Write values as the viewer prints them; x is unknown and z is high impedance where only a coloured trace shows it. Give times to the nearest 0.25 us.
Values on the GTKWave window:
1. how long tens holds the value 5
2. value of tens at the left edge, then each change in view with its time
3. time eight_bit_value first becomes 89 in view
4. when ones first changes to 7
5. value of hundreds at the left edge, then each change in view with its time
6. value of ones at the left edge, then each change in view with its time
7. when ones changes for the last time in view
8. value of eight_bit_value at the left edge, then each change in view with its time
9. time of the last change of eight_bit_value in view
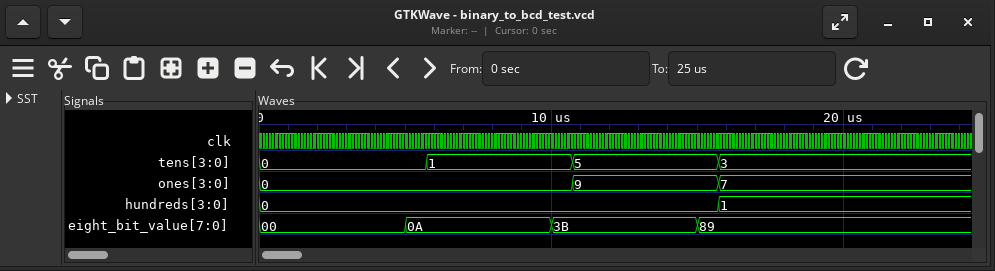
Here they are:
5 us
0, 1 at 5.75 us, 5 at 10.75 us, 3 at 15.75 us
15 us
15.75 us
0, 1 at 15.75 us
0, 9 at 10.75 us, 7 at 15.75 us
15.75 us
00, 0A at 5 us, 3B at 10 us, 89 at 15 us
15 us
